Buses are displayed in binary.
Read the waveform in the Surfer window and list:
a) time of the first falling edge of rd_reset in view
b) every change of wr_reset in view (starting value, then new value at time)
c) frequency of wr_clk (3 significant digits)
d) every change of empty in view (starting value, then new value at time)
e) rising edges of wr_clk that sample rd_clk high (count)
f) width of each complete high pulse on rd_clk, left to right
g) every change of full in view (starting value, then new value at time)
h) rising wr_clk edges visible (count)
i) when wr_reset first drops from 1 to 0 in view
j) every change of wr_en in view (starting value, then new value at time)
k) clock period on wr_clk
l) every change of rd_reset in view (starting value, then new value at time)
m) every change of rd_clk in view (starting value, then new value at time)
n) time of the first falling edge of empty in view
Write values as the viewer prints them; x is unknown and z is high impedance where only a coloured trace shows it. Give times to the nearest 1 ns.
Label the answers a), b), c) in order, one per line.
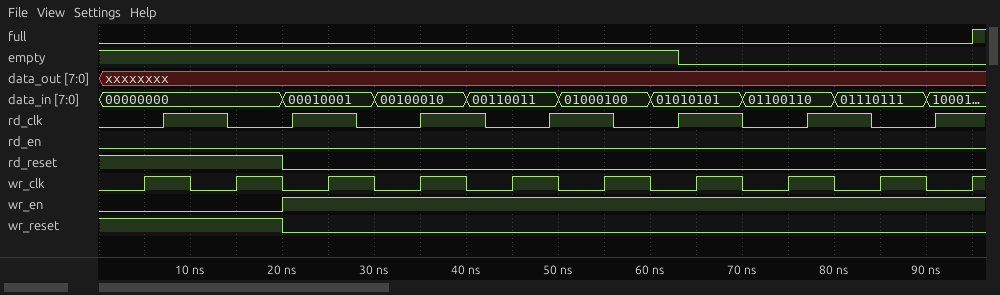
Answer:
a) 20 ns
b) 1, 0 at 20 ns
c) 100 MHz
d) 1, 0 at 63 ns
e) 4
f) 7 ns, 7 ns, 7 ns, 7 ns, 7 ns, 7 ns
g) 0, 1 at 95 ns
h) 10
i) 20 ns
j) 0, 1 at 20 ns
k) 10 ns
l) 1, 0 at 20 ns
m) 0, 1 at 7 ns, 0 at 14 ns, 1 at 21 ns, 0 at 28 ns, 1 at 35 ns, 0 at 42 ns, 1 at 49 ns, 0 at 56 ns, 1 at 63 ns, 0 at 70 ns, 1 at 77 ns, 0 at 84 ns, 1 at 91 ns
n) 63 ns
